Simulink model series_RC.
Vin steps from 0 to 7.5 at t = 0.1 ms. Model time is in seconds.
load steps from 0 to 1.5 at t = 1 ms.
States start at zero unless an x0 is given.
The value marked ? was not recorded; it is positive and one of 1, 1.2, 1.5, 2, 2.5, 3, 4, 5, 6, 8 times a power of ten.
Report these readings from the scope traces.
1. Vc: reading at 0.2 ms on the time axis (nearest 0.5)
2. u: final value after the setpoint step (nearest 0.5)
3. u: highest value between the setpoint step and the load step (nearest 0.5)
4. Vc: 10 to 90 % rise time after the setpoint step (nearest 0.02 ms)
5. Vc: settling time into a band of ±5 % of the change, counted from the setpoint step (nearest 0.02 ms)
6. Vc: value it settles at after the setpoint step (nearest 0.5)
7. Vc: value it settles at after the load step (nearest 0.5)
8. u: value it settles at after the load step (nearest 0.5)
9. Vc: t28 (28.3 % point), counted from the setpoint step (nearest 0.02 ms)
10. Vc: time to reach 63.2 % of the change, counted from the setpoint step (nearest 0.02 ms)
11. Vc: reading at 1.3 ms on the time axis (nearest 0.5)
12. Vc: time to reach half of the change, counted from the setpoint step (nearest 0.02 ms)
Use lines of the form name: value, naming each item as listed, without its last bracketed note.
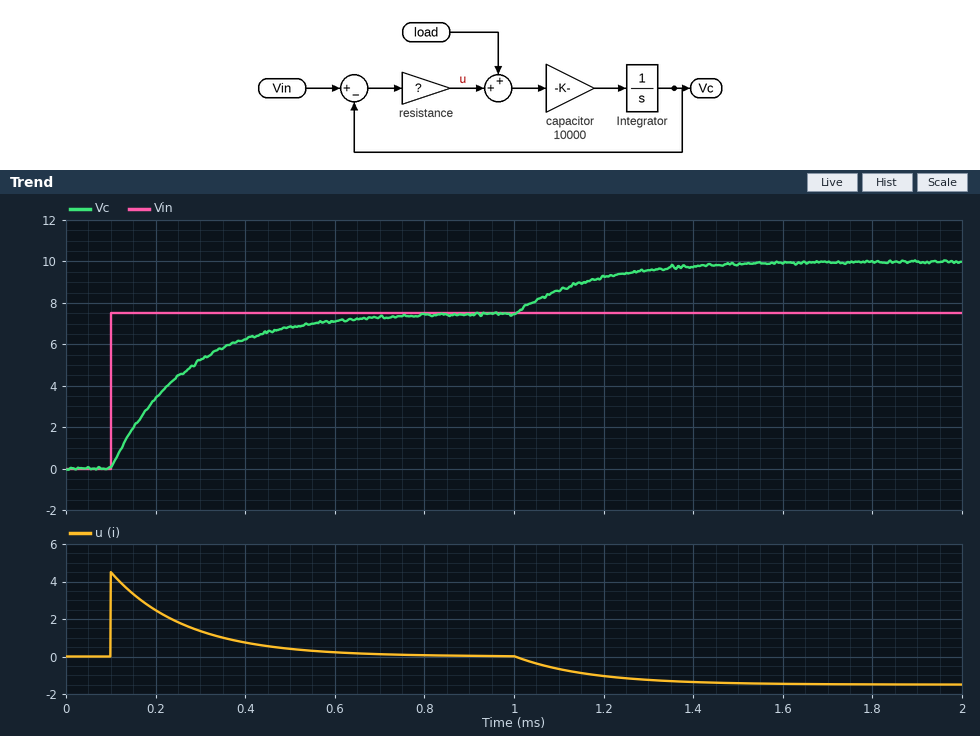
Vc: reading at 0.2 ms on the time axis: 3.5
u: final value after the setpoint step: 0.0
u: highest value between the setpoint step and the load step: 4.5
Vc: 10 to 90 % rise time after the setpoint step: 0.36 ms
Vc: settling time into a band of ±5 % of the change, counted from the setpoint step: 0.50 ms
Vc: value it settles at after the setpoint step: 7.5
Vc: value it settles at after the load step: 10.0
u: value it settles at after the load step: -1.5
Vc: t28 (28.3 % point), counted from the setpoint step: 0.06 ms
Vc: time to reach 63.2 % of the change, counted from the setpoint step: 0.16 ms
Vc: reading at 1.3 ms on the time axis: 9.5
Vc: time to reach half of the change, counted from the setpoint step: 0.12 ms
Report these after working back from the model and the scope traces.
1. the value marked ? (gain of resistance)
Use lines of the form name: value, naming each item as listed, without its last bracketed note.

the value marked ?: 0.6
